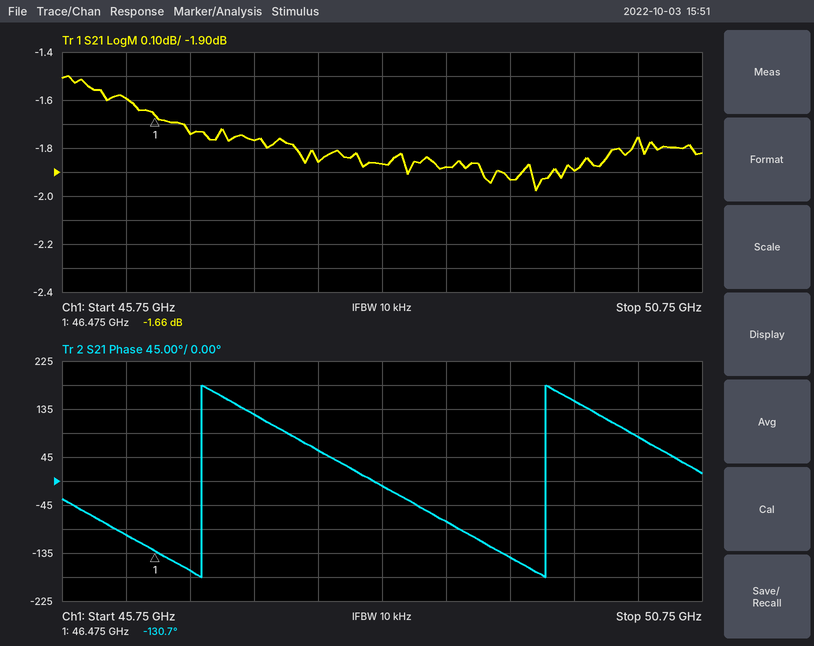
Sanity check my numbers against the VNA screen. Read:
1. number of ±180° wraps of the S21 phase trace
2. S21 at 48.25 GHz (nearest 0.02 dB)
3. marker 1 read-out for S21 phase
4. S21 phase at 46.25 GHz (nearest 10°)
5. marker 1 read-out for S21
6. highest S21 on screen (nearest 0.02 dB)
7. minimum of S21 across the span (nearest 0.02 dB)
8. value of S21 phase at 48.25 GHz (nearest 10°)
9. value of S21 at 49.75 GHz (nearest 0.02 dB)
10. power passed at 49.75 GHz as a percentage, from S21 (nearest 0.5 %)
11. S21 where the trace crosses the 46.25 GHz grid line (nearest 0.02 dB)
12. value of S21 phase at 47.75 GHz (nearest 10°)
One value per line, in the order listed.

2
-1.86 dB
-130.7°
-100°
-1.66 dB
-1.50 dB
-1.98 dB
-10°
-1.90 dB
64.5 %
-1.60 dB
60°
